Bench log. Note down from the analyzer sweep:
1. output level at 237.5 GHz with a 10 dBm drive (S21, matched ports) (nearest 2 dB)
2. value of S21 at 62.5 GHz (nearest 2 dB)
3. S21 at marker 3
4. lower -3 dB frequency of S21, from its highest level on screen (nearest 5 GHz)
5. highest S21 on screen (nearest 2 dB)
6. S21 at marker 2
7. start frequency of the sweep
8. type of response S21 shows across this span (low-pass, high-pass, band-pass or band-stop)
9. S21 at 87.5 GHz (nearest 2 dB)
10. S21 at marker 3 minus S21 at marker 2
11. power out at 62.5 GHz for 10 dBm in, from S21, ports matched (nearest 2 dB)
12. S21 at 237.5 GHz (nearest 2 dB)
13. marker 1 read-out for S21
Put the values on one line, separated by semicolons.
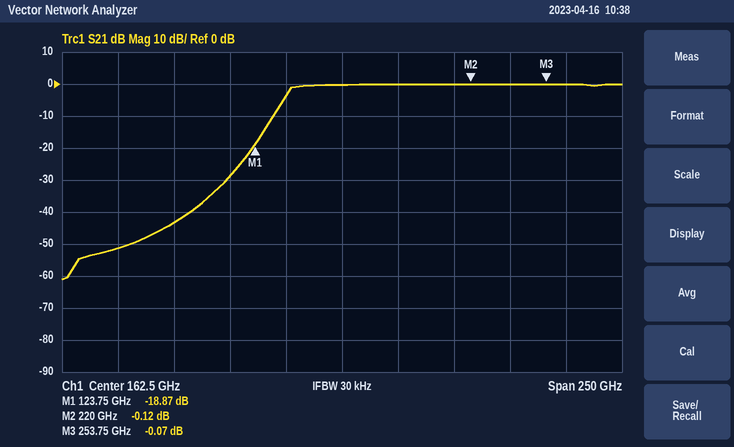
10 dBm; -52 dB; -0.07 dB; 140 GHz; 0 dB; -0.12 dB; 37.5 GHz; high-pass; -44 dB; 0.05 dB; -42 dBm; 0 dB; -18.87 dB
